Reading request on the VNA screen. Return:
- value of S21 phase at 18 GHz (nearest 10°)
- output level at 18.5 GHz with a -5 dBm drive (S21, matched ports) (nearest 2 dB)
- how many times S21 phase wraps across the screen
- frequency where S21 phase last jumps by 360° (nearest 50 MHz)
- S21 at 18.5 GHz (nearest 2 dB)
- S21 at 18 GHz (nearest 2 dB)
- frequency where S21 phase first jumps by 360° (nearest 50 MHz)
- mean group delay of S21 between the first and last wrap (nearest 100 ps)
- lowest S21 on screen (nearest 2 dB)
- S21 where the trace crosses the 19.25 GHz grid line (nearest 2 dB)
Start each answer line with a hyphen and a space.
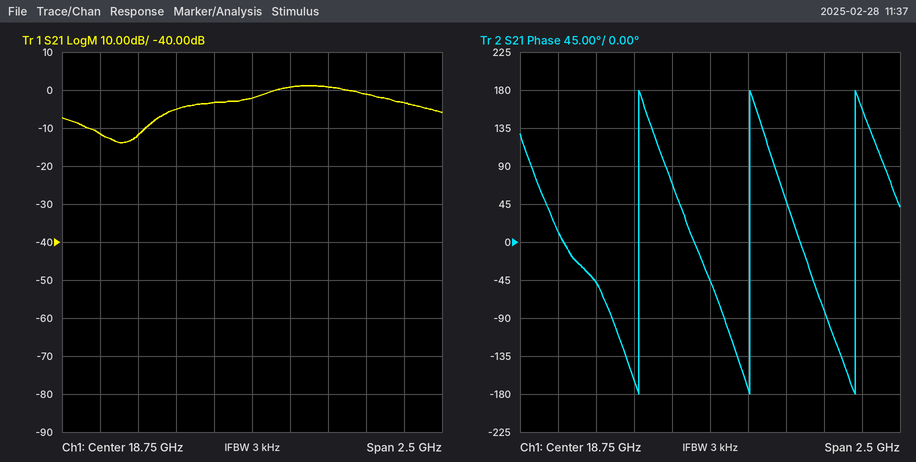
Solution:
- -50°
- -8 dBm
- 3
- 19.70 GHz
- -4 dB
- -12 dB
- 18.30 GHz
- 1.4 ns
- -14 dB
- 0 dB
